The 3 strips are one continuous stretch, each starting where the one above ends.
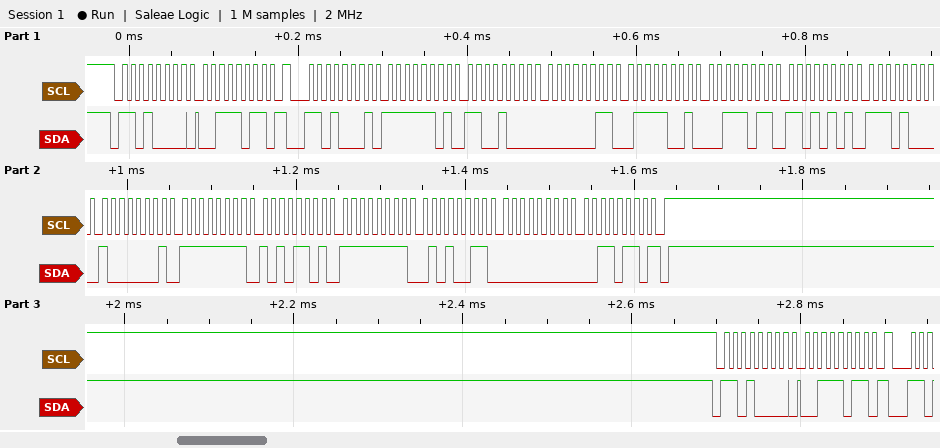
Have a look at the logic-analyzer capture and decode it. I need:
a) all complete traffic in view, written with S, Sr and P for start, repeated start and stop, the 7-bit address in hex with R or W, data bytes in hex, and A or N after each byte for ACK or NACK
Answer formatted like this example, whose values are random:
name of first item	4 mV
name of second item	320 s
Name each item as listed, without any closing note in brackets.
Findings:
all complete traffic in view, written with S, Sr and P for start, repeated start and stop, the 7-bit address in hex with R or W, data bytes in hex, and A or N after each byte for ACK or NACK	S 68W A 3B A Sr 68R A FD A C8 A 03 A 79 A 3B A D5 A E8 A 81 A FF A AD A FF A 53 A 00 A 36 N P S 68W A 3B A
